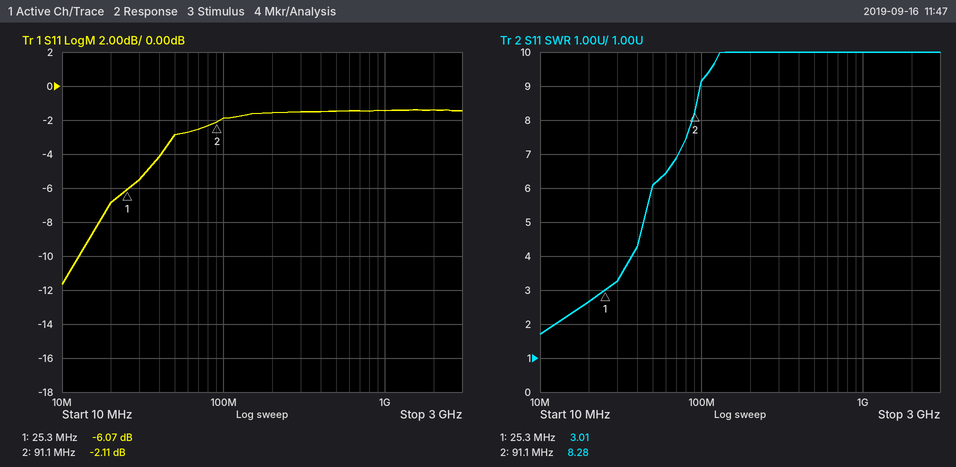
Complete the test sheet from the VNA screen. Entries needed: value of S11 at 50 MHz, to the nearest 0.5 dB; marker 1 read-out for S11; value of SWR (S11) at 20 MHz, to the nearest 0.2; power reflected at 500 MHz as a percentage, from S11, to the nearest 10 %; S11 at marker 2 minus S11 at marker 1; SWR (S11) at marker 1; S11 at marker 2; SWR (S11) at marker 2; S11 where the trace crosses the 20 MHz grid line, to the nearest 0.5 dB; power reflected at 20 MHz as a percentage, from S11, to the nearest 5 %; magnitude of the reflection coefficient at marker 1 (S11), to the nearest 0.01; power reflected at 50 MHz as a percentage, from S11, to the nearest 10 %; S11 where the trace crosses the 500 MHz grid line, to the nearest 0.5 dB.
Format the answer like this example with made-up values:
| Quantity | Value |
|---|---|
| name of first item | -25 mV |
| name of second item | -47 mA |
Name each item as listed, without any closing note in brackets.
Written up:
| Quantity | Value |
|---|---|
| value of S11 at 50 MHz, to the nearest 0.5 dB | -3.0 dB |
| marker 1 read-out for S11 | -6.07 dB |
| value of SWR (S11) at 20 MHz, to the nearest 0.2 | 2.6 |
| power reflected at 500 MHz as a percentage, from S11, to the nearest 10 % | 70 % |
| S11 at marker 2 minus S11 at marker 1 | 3.96 dB |
| SWR (S11) at marker 1 | 3.01 |
| S11 at marker 2 | -2.11 dB |
| SWR (S11) at marker 2 | 8.28 |
| S11 where the trace crosses the 20 MHz grid line, to the nearest 0.5 dB | -7.0 dB |
| power reflected at 20 MHz as a percentage, from S11, to the nearest 5 % | 20 % |
| magnitude of the reflection coefficient at marker 1 (S11), to the nearest 0.01 | 0.50 |
| power reflected at 50 MHz as a percentage, from S11, to the nearest 10 % | 50 % |
| S11 where the trace crosses the 500 MHz grid line, to the nearest 0.5 dB | -1.5 dB |
